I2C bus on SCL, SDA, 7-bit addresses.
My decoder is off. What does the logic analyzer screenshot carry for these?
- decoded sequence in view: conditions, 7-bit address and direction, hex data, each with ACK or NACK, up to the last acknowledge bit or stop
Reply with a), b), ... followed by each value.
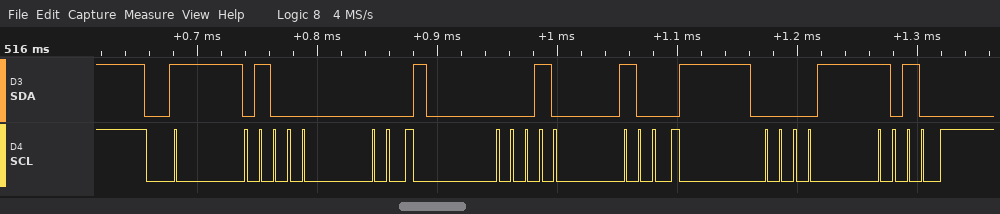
a) start, address 50 write ACK, 14 ACK, 0A ACK
